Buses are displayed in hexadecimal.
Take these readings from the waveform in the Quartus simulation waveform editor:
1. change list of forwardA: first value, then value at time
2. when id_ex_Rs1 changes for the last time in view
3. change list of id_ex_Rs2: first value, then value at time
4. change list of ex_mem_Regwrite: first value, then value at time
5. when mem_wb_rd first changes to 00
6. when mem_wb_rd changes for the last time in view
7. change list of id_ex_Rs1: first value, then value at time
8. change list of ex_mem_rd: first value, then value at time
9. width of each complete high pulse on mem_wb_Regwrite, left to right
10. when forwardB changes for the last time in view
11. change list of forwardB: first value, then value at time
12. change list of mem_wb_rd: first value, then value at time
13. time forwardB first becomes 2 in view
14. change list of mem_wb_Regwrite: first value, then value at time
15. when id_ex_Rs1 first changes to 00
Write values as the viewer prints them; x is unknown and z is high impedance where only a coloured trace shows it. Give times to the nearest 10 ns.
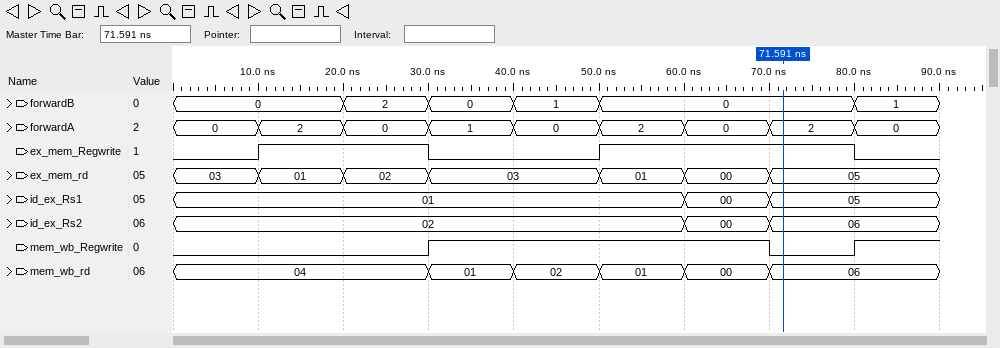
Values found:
0, 2 at 10 ns, 0 at 20 ns, 1 at 30 ns, 0 at 40 ns, 2 at 50 ns, 0 at 60 ns, 2 at 70 ns, 0 at 80 ns
70 ns
02, 00 at 60 ns, 06 at 70 ns
0, 1 at 10 ns, 0 at 30 ns, 1 at 50 ns, 0 at 80 ns
60 ns
70 ns
01, 00 at 60 ns, 05 at 70 ns
03, 01 at 10 ns, 02 at 20 ns, 03 at 30 ns, 01 at 50 ns, 00 at 60 ns, 05 at 70 ns
40 ns
80 ns
0, 2 at 20 ns, 0 at 30 ns, 1 at 40 ns, 0 at 50 ns, 1 at 80 ns
04, 01 at 30 ns, 02 at 40 ns, 01 at 50 ns, 00 at 60 ns, 06 at 70 ns
20 ns
0, 1 at 30 ns, 0 at 70 ns, 1 at 80 ns
60 ns
